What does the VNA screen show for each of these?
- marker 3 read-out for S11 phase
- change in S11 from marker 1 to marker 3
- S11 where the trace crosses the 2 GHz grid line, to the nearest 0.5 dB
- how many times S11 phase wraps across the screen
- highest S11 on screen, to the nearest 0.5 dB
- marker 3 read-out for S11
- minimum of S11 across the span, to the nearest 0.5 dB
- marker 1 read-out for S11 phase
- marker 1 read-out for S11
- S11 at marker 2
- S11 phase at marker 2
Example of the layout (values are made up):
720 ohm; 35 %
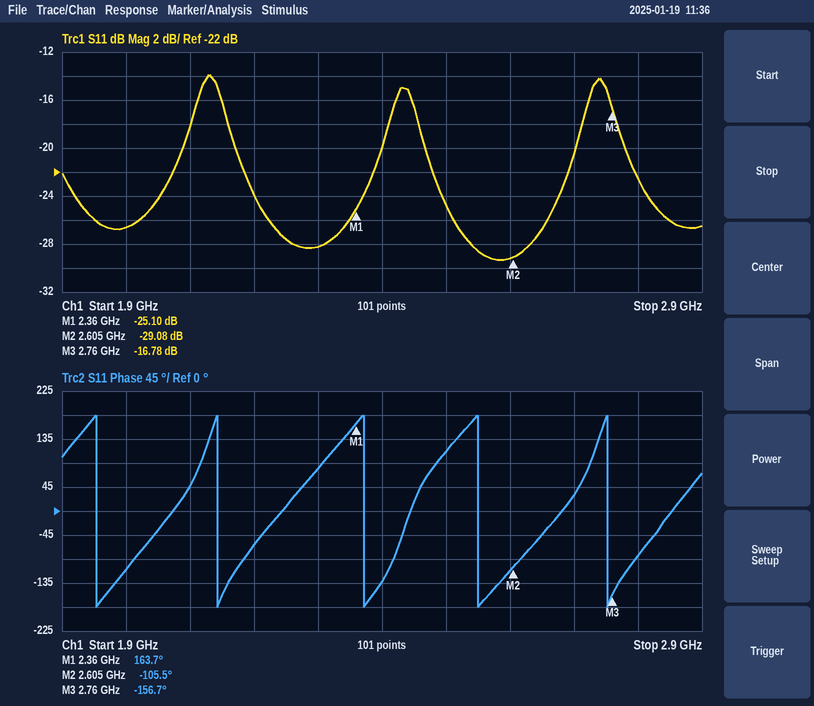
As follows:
-156.7°; 8.32 dB; -26.5 dB; 5; -14.0 dB; -16.78 dB; -29.5 dB; 163.7°; -25.10 dB; -29.08 dB; -105.5°
